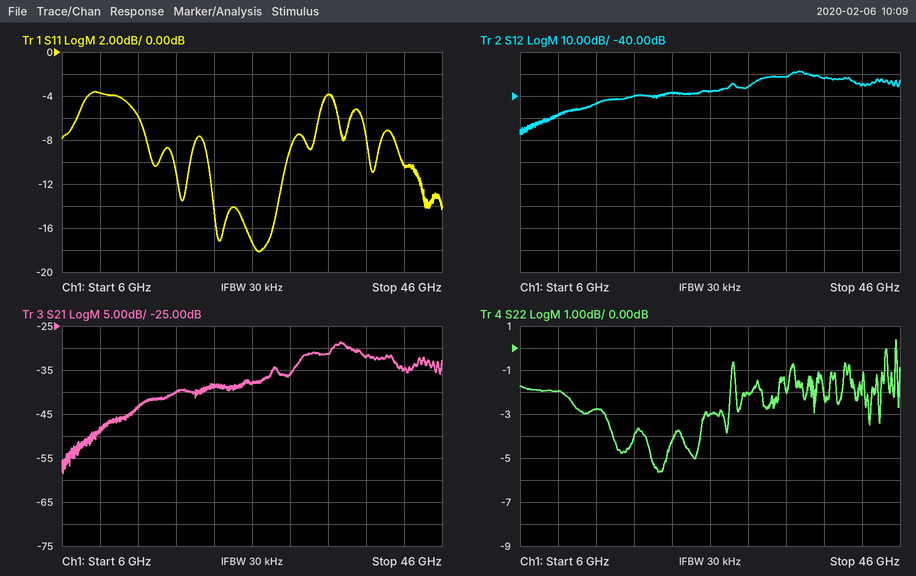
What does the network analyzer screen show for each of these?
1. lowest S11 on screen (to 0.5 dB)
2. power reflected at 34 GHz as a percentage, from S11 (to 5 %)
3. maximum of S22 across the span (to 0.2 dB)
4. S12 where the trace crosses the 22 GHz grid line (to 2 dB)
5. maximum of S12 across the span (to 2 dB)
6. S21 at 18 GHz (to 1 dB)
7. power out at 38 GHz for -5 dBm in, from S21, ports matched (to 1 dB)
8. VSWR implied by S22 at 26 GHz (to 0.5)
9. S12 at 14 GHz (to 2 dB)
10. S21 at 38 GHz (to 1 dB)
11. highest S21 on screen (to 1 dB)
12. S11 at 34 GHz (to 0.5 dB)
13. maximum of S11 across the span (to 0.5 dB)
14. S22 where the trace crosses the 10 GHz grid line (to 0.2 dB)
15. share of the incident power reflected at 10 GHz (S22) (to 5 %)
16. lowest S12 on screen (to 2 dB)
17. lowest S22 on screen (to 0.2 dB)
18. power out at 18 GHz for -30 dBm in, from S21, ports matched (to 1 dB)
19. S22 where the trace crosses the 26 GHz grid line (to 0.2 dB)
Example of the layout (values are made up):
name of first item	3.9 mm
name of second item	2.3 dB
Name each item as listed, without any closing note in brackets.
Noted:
lowest S11 on screen	-18.0 dB
power reflected at 34 GHz as a percentage, from S11	40 %
maximum of S22 across the span	0.4 dB
S12 where the trace crosses the 22 GHz grid line	-38 dB
maximum of S12 across the span	-28 dB
S21 at 18 GHz	-40 dB
power out at 38 GHz for -5 dBm in, from S21, ports matched	-37 dBm
VSWR implied by S22 at 26 GHz	6.0
S12 at 14 GHz	-44 dB
S21 at 38 GHz	-32 dB
highest S21 on screen	-29 dB
S11 at 34 GHz	-4.0 dB
maximum of S11 across the span	-3.5 dB
S22 where the trace crosses the 10 GHz grid line	-2.0 dB
share of the incident power reflected at 10 GHz (S22)	65 %
lowest S12 on screen	-58 dB
lowest S22 on screen	-5.6 dB
power out at 18 GHz for -30 dBm in, from S21, ports matched	-70 dBm
S22 where the trace crosses the 26 GHz grid line	-3.0 dB
